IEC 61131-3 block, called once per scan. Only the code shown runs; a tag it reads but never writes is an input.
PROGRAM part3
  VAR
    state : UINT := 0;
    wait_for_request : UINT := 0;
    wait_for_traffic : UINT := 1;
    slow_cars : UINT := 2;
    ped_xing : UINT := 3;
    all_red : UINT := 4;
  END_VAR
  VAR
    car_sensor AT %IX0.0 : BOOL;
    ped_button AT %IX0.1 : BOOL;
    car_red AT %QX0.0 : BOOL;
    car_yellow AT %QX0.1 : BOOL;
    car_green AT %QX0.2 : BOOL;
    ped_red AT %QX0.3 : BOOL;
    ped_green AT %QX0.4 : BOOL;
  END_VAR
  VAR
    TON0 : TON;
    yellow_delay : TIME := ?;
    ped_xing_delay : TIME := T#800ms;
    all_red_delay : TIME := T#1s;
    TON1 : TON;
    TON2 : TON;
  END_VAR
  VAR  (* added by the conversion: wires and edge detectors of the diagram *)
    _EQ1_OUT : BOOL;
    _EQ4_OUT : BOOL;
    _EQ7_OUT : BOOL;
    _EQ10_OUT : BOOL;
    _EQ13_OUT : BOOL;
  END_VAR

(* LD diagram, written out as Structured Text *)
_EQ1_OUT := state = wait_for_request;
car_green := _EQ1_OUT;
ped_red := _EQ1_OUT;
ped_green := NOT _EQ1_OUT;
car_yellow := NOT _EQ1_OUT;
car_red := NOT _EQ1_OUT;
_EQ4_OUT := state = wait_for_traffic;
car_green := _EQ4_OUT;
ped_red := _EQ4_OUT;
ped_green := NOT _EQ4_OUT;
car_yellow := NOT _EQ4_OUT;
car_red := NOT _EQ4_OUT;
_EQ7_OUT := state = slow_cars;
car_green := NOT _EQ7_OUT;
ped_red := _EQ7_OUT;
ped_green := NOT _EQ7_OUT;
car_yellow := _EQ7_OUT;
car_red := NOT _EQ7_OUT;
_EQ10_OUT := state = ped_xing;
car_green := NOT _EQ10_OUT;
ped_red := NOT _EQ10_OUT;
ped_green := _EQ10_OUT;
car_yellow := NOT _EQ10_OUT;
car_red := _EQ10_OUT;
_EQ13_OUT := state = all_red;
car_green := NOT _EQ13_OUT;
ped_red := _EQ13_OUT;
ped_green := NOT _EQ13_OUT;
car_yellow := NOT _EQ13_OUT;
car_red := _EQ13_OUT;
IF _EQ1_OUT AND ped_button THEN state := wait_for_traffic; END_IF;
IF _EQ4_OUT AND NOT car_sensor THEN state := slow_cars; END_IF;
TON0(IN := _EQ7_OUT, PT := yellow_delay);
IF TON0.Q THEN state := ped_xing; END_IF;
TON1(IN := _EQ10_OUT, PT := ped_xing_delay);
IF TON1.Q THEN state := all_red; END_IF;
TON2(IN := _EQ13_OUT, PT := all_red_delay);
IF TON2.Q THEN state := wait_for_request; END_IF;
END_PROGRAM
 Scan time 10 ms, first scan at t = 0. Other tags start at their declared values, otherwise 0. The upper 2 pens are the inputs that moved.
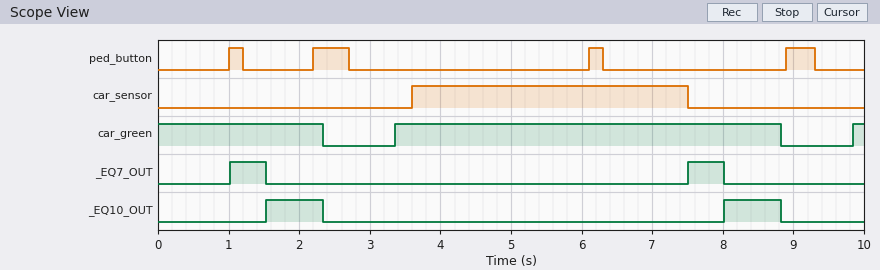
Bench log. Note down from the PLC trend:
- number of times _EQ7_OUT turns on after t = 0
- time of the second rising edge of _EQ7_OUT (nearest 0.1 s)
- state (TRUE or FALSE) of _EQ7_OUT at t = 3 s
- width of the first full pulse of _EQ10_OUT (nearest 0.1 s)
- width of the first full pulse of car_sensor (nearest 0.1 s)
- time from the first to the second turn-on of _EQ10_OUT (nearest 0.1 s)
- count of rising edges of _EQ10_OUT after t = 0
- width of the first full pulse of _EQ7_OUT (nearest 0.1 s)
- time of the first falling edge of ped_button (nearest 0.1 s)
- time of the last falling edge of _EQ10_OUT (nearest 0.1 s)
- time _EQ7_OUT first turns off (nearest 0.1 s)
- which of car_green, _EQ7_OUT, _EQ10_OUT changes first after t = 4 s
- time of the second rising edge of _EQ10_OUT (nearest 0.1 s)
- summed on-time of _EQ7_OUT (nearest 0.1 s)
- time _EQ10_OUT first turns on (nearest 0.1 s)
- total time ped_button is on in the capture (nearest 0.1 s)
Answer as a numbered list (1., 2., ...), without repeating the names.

1. 2
2. 7.5 s
3. FALSE
4. 0.8 s
5. 3.9 s
6. 6.5 s
7. 2
8. 0.5 s
9. 1.2 s
10. 8.8 s
11. 1.5 s
12. _EQ7_OUT
13. 8.0 s
14. 1.0 s
15. 1.5 s
16. 1.3 s
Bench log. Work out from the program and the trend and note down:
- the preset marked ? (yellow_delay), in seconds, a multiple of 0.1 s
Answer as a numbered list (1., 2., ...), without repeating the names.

1. 0.5 s
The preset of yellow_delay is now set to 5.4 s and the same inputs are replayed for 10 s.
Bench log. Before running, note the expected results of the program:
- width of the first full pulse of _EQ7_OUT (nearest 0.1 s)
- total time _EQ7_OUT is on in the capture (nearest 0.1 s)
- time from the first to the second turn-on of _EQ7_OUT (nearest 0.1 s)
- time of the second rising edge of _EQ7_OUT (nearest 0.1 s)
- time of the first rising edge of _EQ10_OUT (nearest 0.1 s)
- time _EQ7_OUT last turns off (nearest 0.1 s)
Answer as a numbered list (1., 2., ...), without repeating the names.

1. 5.4 s
2. 6.5 s
3. 7.9 s
4. 8.9 s
5. 6.4 s
6. 6.4 s
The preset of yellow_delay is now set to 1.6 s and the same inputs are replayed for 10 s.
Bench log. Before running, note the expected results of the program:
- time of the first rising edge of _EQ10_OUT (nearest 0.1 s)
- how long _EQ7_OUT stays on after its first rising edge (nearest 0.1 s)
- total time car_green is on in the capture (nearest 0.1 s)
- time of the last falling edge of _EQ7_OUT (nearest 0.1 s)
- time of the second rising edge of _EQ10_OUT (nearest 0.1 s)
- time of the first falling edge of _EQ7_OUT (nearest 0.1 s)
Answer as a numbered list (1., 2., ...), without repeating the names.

1. 2.6 s
2. 1.6 s
3. 8.9 s
4. 9.1 s
5. 9.1 s
6. 2.6 s
